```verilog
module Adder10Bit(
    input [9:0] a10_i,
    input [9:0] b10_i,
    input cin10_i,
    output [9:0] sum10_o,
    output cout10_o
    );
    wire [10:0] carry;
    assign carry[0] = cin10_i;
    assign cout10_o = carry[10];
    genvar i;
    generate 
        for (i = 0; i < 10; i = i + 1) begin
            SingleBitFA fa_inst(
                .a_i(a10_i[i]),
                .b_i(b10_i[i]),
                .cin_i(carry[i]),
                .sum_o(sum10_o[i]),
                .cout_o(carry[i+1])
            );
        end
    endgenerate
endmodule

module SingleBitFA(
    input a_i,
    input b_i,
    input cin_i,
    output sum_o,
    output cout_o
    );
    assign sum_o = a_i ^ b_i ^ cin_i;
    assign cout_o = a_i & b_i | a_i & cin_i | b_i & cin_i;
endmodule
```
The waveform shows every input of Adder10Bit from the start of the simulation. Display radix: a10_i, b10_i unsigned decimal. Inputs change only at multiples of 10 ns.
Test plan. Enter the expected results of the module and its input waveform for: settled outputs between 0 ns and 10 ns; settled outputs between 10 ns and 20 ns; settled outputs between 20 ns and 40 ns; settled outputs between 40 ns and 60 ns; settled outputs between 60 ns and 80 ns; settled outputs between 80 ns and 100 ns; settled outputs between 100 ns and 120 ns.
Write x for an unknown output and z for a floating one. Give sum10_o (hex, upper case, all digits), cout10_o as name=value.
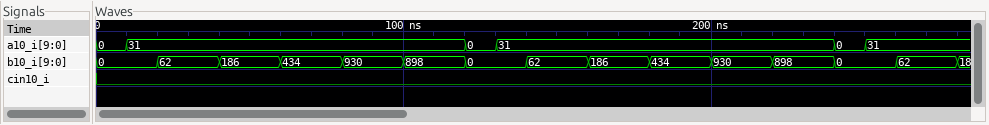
sum10_o=000, cout10_o=0
sum10_o=01F, cout10_o=0
sum10_o=05D, cout10_o=0
sum10_o=0D9, cout10_o=0
sum10_o=1D1, cout10_o=0
sum10_o=3C1, cout10_o=0
sum10_o=3A1, cout10_o=0
